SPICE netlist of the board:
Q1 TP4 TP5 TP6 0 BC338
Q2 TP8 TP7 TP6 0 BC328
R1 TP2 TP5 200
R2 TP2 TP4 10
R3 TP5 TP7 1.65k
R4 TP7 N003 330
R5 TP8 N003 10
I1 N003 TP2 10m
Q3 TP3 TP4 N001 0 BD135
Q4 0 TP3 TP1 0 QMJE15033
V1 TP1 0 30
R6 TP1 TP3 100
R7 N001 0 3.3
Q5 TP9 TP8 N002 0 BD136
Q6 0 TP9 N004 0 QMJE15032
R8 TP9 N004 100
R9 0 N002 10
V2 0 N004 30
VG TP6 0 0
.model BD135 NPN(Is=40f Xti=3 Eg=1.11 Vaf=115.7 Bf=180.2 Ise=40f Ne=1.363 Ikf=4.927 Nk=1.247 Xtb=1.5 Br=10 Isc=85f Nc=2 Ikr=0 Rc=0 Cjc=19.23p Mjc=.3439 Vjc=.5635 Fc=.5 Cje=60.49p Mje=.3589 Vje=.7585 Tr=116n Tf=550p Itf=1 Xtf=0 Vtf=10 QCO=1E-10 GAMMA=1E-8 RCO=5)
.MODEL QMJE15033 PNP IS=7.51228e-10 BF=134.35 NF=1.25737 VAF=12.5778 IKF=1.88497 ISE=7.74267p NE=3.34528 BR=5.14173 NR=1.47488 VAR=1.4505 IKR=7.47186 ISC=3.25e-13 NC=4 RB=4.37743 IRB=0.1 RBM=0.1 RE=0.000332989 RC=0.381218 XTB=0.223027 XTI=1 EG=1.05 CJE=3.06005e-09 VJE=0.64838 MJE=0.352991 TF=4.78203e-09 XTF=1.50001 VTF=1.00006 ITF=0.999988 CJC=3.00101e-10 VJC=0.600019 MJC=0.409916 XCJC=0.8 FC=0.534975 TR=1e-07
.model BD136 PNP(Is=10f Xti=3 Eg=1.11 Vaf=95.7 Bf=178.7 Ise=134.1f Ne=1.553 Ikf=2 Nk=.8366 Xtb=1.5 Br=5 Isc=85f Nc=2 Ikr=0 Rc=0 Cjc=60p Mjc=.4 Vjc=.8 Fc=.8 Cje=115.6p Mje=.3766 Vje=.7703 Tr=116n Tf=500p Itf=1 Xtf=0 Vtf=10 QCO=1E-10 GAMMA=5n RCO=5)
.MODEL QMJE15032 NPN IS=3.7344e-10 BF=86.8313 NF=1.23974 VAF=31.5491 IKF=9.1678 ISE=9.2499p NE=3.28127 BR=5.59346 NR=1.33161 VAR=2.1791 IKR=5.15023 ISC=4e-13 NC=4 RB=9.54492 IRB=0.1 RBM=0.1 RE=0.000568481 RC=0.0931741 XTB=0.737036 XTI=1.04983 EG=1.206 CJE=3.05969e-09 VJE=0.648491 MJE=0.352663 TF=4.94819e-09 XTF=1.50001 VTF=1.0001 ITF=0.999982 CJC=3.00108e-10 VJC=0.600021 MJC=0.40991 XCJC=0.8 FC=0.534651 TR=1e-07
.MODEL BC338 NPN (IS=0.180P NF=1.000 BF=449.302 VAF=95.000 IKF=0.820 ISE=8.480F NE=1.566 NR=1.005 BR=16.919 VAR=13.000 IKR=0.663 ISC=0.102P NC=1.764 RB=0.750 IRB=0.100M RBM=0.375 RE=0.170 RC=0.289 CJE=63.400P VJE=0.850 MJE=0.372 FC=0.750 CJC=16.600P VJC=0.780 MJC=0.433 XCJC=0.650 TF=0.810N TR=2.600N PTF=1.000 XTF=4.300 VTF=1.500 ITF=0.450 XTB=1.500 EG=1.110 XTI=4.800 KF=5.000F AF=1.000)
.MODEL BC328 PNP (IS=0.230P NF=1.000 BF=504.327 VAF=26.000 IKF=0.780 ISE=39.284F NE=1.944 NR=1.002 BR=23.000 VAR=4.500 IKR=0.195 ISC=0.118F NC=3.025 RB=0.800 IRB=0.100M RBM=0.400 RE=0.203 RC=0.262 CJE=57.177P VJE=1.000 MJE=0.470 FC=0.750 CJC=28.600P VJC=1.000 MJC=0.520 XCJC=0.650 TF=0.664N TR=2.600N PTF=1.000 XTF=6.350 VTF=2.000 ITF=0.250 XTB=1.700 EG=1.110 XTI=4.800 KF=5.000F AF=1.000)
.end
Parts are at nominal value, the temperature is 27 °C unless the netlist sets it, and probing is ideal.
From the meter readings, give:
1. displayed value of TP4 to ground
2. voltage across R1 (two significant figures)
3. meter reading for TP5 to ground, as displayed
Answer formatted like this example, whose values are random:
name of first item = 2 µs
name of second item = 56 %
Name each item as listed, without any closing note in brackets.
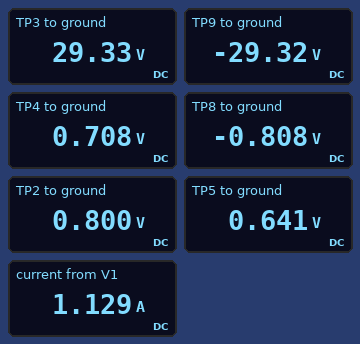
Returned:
displayed value of TP4 to ground = 0.708 V
voltage across R1 = 160 mV
meter reading for TP5 to ground, as displayed = 0.641 V
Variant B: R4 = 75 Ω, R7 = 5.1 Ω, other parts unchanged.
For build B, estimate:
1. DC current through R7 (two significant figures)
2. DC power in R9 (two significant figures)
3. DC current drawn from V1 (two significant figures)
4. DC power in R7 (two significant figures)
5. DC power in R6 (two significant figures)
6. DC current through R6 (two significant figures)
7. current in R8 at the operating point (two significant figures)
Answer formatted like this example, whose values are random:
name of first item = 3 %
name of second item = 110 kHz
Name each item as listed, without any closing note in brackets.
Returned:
DC current through R7 = 8.0 mA
DC power in R9 = 320 nW
DC current drawn from V1 = 560 mA
DC power in R7 = 330 µW
DC power in R6 = 4.1 mW
DC current through R6 = 6.4 mA
current in R8 at the operating point = 180 µA
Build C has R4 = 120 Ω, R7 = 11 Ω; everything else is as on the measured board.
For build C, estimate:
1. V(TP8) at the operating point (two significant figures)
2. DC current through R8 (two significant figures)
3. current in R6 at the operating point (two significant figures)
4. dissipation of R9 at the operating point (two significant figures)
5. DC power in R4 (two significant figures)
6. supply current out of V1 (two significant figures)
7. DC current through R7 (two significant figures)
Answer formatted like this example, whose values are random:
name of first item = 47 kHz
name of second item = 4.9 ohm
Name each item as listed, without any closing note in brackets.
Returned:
V(TP8) at the operating point = -640 mV
DC current through R8 = 600 µA
current in R6 at the operating point = 4.8 mA
dissipation of R9 at the operating point = 3.7 µW
DC power in R4 = 76 µW
supply current out of V1 = 11 mA
DC current through R7 = 4.9 mA
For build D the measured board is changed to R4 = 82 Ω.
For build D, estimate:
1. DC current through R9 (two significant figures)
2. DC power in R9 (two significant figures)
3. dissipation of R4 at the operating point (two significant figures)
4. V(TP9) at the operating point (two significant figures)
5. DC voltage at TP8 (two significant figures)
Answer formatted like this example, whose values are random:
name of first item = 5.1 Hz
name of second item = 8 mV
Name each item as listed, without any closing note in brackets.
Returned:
DC current through R9 = 220 µA
DC power in R9 = 480 nW
dissipation of R4 at the operating point = 52 µW
V(TP9) at the operating point = -30 V
DC voltage at TP8 = -610 mV
